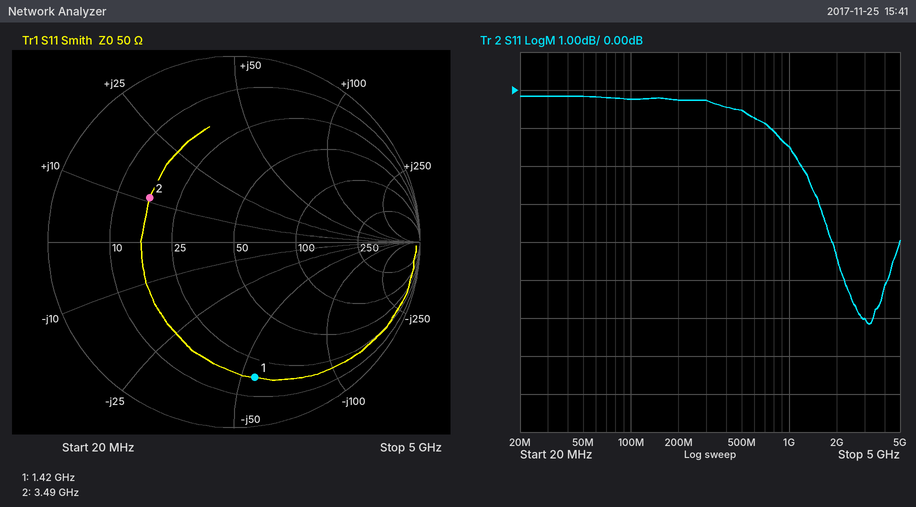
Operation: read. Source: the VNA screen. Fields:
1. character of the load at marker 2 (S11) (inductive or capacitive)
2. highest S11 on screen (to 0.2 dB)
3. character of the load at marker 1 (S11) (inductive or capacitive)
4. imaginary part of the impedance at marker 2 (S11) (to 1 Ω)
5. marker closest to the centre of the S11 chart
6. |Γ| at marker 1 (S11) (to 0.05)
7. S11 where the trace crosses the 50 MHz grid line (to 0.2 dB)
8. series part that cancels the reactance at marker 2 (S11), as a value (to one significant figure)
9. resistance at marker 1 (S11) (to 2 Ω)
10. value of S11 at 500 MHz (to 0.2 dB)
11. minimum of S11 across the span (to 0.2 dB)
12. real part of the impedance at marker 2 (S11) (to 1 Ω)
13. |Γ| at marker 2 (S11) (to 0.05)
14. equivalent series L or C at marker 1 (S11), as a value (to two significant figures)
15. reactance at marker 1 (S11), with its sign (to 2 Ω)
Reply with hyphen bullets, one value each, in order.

- inductive
- -0.2 dB
- capacitive
- +11 Ω
- marker 2
- 0.75
- -0.2 dB
- 4 pF
- 18 Ω
- -0.6 dB
- -6.2 dB
- 17 Ω
- 0.50
- 2.0 pF
- -56 Ω
